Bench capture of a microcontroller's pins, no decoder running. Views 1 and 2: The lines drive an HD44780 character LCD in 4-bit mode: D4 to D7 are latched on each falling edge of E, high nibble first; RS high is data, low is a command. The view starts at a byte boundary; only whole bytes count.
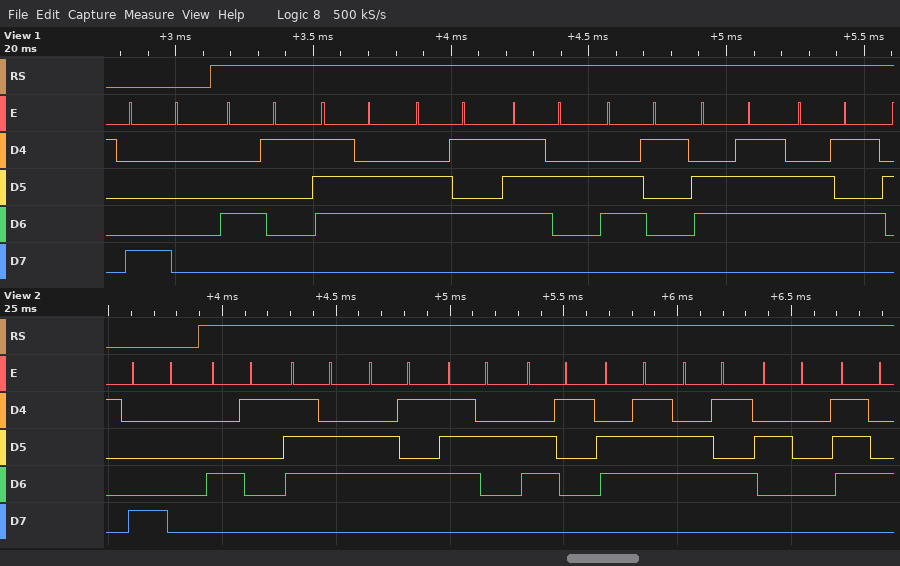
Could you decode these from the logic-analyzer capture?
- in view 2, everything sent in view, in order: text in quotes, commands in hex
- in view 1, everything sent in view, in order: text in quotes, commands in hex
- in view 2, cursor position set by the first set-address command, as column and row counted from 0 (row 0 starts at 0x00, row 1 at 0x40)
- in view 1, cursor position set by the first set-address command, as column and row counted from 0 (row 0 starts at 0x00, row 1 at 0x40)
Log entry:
0x80 "Average t"
0x80 "Average"
column 0, row 0
column 0, row 0
